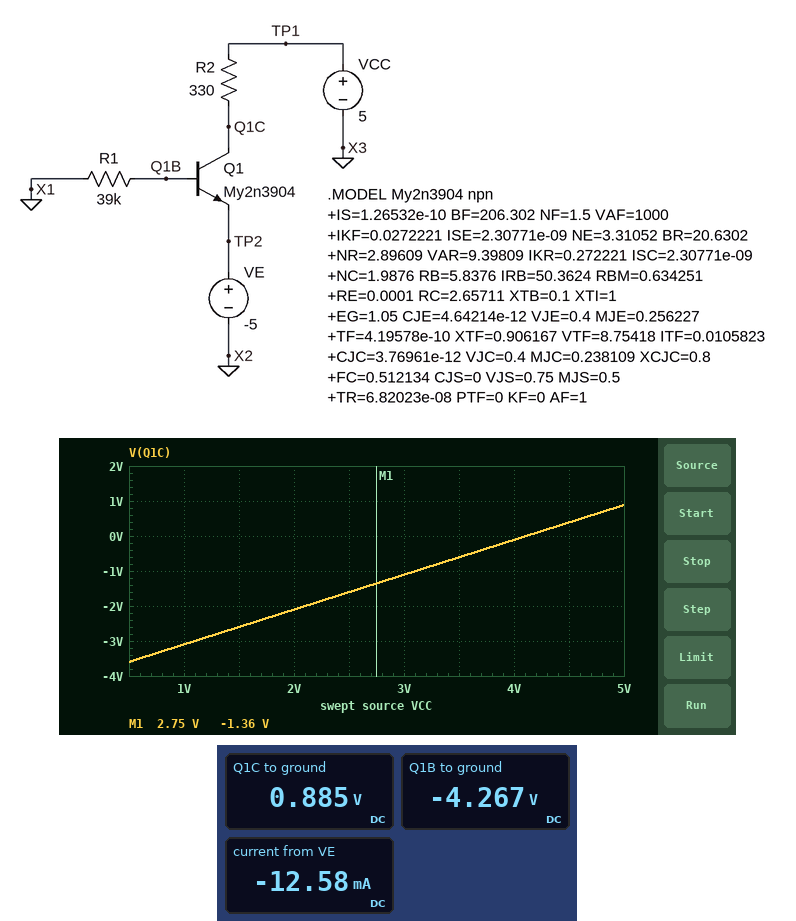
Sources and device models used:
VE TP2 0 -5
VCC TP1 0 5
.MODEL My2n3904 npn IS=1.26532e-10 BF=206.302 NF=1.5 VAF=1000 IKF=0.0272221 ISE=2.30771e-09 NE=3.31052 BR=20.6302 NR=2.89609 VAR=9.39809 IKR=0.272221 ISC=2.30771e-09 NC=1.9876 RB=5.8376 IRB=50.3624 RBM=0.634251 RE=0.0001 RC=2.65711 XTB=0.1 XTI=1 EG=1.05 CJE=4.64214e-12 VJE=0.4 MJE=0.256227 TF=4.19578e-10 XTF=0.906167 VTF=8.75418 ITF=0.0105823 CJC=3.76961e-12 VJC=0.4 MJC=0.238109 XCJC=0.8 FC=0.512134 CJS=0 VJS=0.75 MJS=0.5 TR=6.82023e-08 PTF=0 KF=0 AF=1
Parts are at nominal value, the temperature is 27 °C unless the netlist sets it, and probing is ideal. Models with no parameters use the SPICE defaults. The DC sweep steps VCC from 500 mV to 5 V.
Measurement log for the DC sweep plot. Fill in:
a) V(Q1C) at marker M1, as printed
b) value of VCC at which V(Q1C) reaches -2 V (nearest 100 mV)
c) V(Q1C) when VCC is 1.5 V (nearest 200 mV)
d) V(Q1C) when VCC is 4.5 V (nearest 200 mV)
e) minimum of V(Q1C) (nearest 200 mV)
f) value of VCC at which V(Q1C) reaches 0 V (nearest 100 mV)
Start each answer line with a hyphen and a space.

- -1.36 V
- 2.1 V
- -2.6 V
- 400 mV
- -3.6 V
- 4.1 V
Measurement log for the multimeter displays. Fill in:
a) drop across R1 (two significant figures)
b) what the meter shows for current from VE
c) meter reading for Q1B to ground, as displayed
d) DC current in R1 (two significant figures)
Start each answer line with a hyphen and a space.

- 4.3 V
- -12.58 mA
- -4.267 V
- 110 µA
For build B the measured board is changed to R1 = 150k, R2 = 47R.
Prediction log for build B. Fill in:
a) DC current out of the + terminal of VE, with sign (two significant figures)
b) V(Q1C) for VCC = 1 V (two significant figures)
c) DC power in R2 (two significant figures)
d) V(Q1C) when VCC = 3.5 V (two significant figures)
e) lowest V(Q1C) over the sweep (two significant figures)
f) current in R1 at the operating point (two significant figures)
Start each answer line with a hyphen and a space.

- -3.8 mA
- 820 mV
- 680 µW
- 3.3 V
- 320 mV
- 29 µA
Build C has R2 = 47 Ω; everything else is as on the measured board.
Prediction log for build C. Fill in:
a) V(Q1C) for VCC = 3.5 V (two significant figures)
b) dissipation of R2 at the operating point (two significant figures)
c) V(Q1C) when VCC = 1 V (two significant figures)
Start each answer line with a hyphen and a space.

- 2.9 V
- 7.4 mW
- 410 mV
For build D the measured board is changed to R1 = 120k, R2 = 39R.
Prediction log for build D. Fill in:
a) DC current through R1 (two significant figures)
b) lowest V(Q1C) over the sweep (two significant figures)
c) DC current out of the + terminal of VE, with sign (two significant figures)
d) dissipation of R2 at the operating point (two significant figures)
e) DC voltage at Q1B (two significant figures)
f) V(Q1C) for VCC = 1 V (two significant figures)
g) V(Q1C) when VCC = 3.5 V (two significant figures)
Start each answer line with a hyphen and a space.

- 36 µA
- 320 mV
- -4.8 mA
- 870 µW
- -4.3 V
- 820 mV
- 3.3 V
